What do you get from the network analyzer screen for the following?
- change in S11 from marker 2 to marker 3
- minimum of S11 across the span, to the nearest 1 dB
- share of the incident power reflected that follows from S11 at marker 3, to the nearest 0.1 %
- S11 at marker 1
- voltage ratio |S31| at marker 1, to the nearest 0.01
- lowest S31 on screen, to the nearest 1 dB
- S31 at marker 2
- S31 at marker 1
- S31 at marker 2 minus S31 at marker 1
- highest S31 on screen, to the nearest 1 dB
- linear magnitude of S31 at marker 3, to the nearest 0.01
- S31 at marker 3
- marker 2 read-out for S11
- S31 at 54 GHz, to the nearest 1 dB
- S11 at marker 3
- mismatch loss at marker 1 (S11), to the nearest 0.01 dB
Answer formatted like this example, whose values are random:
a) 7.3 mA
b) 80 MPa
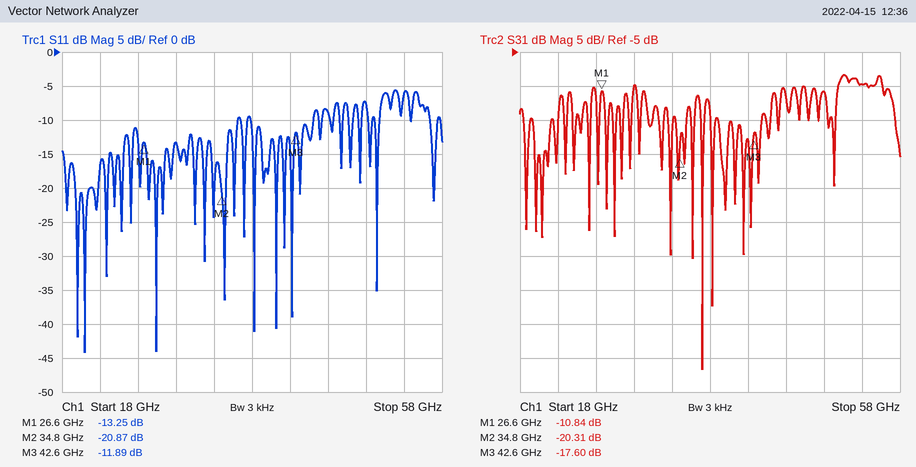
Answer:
a) 8.98 dB
b) -44 dB
c) 6.5 %
d) -13.25 dB
e) 0.29
f) -52 dB
g) -20.31 dB
h) -10.84 dB
i) -9.47 dB
j) -8 dB
k) 0.13
l) -17.60 dB
m) -20.87 dB
n) -10 dB
o) -11.89 dB
p) 0.21 dB
